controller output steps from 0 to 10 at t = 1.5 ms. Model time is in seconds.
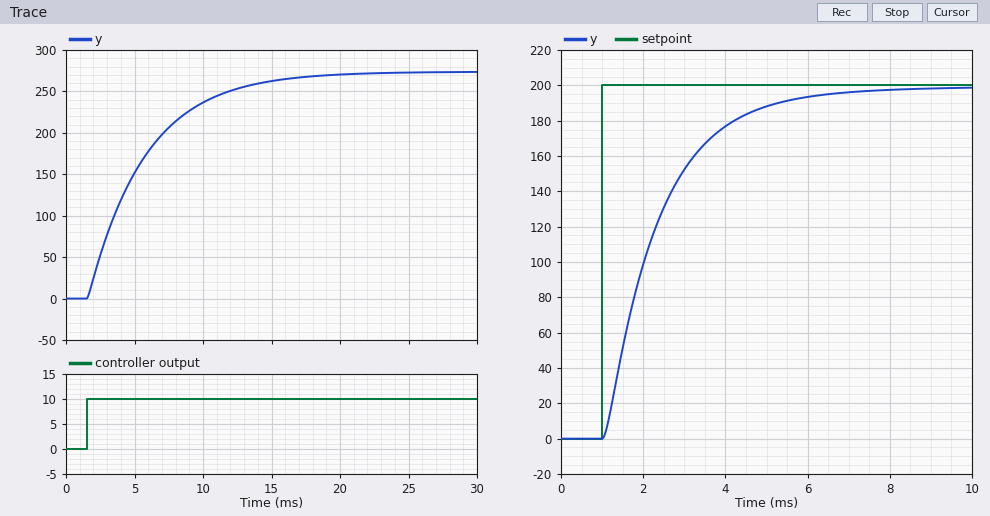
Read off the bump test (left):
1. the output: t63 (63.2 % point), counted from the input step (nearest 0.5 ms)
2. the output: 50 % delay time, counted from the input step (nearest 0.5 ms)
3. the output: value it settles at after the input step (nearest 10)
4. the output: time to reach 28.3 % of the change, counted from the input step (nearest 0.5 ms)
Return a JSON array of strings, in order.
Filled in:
["4.5 ms", "3.0 ms", "270", "1.5 ms"]
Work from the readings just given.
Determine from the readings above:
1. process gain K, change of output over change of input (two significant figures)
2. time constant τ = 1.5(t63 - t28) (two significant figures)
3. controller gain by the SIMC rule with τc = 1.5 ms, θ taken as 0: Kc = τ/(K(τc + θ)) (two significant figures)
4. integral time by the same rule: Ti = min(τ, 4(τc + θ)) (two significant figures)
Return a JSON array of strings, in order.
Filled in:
["27", "4.5 ms", "0.11", "4.5 ms"]
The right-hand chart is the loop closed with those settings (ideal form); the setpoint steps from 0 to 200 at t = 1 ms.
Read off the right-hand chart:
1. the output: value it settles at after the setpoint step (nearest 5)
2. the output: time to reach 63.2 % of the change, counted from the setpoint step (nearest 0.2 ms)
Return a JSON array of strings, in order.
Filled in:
["200", "1.4 ms"]
